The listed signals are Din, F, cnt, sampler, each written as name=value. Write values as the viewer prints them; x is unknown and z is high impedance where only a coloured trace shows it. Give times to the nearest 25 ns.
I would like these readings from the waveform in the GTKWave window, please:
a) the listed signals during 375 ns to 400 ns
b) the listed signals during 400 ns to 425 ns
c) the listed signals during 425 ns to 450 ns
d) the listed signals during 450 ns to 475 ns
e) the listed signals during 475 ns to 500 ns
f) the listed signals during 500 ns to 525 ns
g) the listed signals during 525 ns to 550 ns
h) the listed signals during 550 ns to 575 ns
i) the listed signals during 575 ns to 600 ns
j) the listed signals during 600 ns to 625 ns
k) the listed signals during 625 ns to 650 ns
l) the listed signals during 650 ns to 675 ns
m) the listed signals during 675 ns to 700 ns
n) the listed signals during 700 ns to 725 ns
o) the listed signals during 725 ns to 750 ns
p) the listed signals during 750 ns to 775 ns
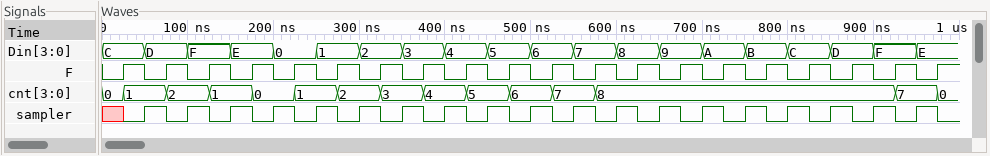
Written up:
Din=3, F=1, cnt=4, sampler=0
Din=4, F=0, cnt=4, sampler=1
Din=4, F=1, cnt=5, sampler=0
Din=5, F=0, cnt=5, sampler=1
Din=5, F=1, cnt=6, sampler=0
Din=6, F=0, cnt=6, sampler=1
Din=6, F=1, cnt=7, sampler=0
Din=7, F=0, cnt=7, sampler=1
Din=7, F=1, cnt=8, sampler=0
Din=8, F=0, cnt=8, sampler=1
Din=8, F=1, cnt=8, sampler=0
Din=9, F=0, cnt=8, sampler=1
Din=9, F=1, cnt=8, sampler=0
Din=A, F=0, cnt=8, sampler=1
Din=A, F=1, cnt=8, sampler=0
Din=B, F=0, cnt=8, sampler=1
